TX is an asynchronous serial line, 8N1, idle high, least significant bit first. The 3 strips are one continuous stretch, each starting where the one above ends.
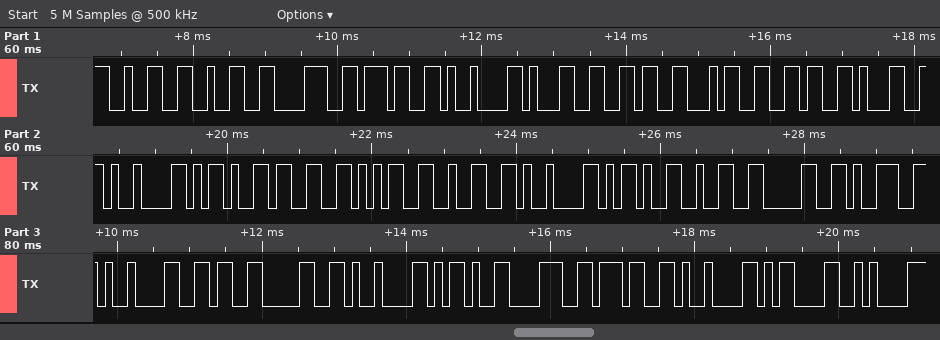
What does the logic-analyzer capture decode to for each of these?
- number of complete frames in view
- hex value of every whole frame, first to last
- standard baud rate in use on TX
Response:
30
32 32 38 37 09 31 36 34 36 31 09 2D 33 35 32 09 2D 32 30 39 09 36 30 09 2D 38 37 09 0D 0A
9600 baud
